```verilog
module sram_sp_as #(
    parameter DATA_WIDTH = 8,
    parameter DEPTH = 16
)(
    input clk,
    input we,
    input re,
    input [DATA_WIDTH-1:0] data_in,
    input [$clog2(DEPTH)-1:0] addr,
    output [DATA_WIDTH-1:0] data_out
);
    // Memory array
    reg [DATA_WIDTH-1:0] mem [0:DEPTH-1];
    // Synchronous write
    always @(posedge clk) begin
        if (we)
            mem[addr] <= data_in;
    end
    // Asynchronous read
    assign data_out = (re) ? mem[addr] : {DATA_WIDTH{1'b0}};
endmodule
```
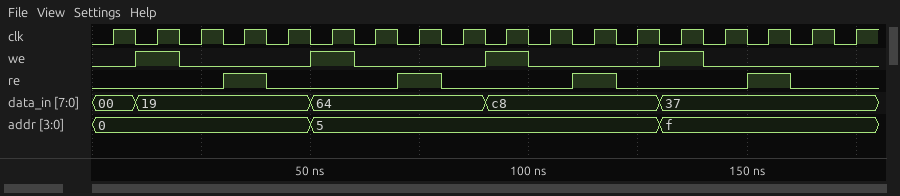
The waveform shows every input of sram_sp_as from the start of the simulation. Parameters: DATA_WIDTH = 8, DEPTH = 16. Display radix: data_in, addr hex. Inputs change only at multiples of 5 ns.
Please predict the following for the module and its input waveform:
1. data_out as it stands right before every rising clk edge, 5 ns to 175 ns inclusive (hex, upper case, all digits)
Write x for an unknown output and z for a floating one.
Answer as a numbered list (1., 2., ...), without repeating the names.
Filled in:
1. 00, 00, 00, 19, 00, 00, 00, 64, 00, 00, 00, C8, 00, 00, 00, 37, 00, 00
